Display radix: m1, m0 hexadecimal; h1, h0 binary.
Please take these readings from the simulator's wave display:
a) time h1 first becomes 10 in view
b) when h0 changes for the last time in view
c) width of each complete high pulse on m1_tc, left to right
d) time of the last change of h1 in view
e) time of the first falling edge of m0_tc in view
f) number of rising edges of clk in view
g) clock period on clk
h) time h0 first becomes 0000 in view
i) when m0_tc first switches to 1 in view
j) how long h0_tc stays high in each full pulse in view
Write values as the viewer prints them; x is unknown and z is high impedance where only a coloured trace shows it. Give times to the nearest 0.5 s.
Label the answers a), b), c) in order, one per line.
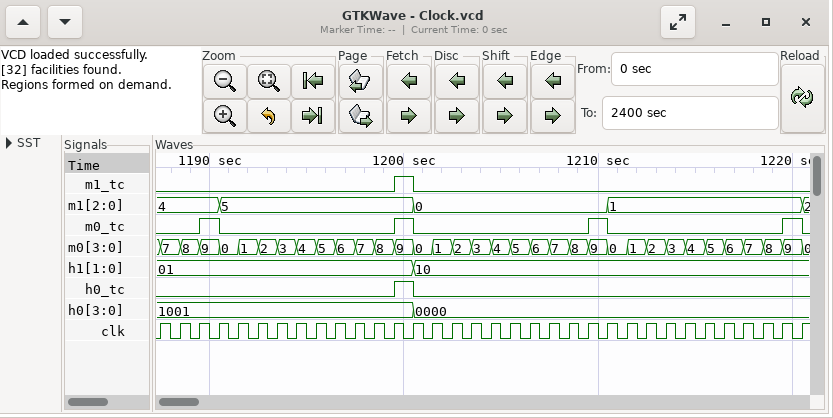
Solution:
a) 1200.5 s
b) 1200.5 s
c) 1 s
d) 1200.5 s
e) 1190.5 s
f) 34
g) 1 s
h) 1200.5 s
i) 1189.5 s
j) 1 s
